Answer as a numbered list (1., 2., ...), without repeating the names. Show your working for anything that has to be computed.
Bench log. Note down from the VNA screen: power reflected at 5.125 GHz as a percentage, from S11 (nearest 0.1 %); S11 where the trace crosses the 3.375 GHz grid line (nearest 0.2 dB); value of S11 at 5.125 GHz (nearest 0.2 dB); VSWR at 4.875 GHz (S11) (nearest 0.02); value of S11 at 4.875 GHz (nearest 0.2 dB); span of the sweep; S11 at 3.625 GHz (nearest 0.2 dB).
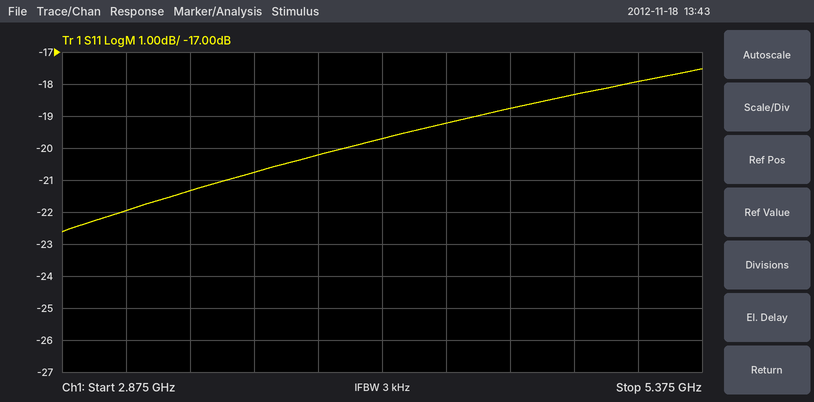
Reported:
1. 10^(-18/10) ≈ 1.6 %
2. -21.4 dB
3. -18.0 dB
4. |Γ| = 10^(-18.4/20) = 0.1202; VSWR = (1 + 0.1202)/(1 − 0.1202) ≈ 1.27, so 1.28 to the nearest 0.02
5. -18.4 dB
6. 2.5 GHz
7. -20.8 dB
